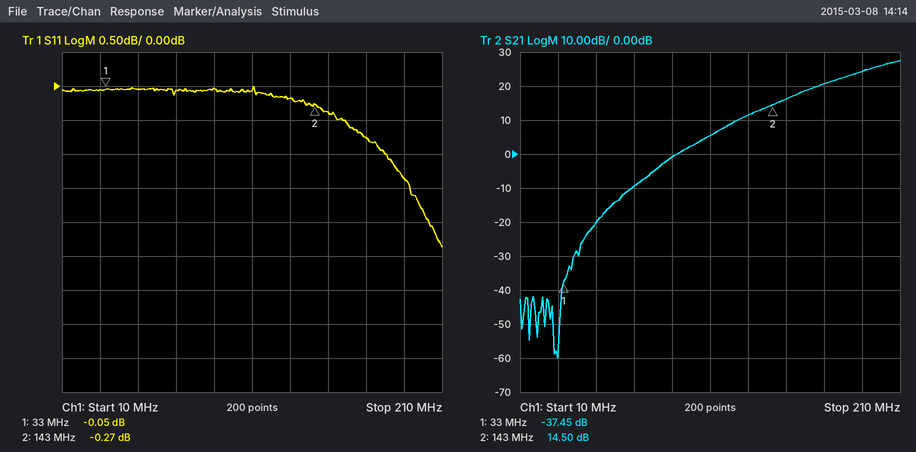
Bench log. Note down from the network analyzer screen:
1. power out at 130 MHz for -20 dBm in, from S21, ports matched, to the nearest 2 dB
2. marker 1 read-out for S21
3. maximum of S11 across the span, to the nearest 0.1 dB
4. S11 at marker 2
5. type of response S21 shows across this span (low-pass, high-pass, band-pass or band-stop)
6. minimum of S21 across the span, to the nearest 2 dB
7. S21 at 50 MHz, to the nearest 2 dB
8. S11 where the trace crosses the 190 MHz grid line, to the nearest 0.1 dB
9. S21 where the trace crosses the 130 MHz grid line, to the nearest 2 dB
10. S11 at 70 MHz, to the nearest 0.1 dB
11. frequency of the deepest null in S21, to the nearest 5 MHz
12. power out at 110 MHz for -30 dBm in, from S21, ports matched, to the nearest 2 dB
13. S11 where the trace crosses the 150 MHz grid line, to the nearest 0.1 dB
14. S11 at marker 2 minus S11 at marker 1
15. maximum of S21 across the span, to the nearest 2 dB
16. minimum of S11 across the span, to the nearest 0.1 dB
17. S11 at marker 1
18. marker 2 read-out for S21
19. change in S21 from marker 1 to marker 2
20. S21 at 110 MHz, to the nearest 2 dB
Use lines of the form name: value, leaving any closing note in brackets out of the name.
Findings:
power out at 130 MHz for -20 dBm in, from S21, ports matched, to the nearest 2 dB: -8 dBm
marker 1 read-out for S21: -37.45 dB
maximum of S11 across the span, to the nearest 0.1 dB: 0.0 dB
S11 at marker 2: -0.27 dB
type of response S21 shows across this span: high-pass
minimum of S21 across the span, to the nearest 2 dB: -60 dB
S21 at 50 MHz, to the nearest 2 dB: -20 dB
S11 where the trace crosses the 190 MHz grid line, to the nearest 0.1 dB: -1.4 dB
S21 where the trace crosses the 130 MHz grid line, to the nearest 2 dB: 12 dB
S11 at 70 MHz, to the nearest 0.1 dB: -0.1 dB
frequency of the deepest null in S21, to the nearest 5 MHz: 30 MHz
power out at 110 MHz for -30 dBm in, from S21, ports matched, to the nearest 2 dB: -24 dBm
S11 where the trace crosses the 150 MHz grid line, to the nearest 0.1 dB: -0.4 dB
S11 at marker 2 minus S11 at marker 1: -0.22 dB
maximum of S21 across the span, to the nearest 2 dB: 28 dB
minimum of S11 across the span, to the nearest 0.1 dB: -2.4 dB
S11 at marker 1: -0.05 dB
marker 2 read-out for S21: 14.50 dB
change in S21 from marker 1 to marker 2: 51.95 dB
S21 at 110 MHz, to the nearest 2 dB: 6 dB
